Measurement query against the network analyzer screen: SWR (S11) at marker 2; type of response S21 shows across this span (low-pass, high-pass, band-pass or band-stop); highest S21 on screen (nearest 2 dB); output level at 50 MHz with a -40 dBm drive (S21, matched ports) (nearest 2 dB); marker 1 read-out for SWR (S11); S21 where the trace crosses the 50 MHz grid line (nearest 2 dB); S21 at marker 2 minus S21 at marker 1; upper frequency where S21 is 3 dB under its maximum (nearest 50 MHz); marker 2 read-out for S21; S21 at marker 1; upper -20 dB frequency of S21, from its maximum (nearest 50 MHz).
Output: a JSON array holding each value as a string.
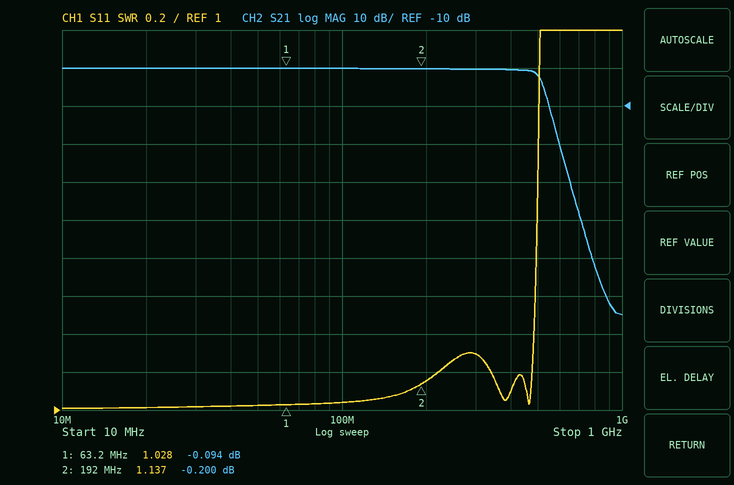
["1.137", "low-pass", "0 dB", "-40 dBm", "1.028", "0 dB", "-0.106 dB", "500 MHz", "-0.200 dB", "-0.094 dB", "600 MHz"]
